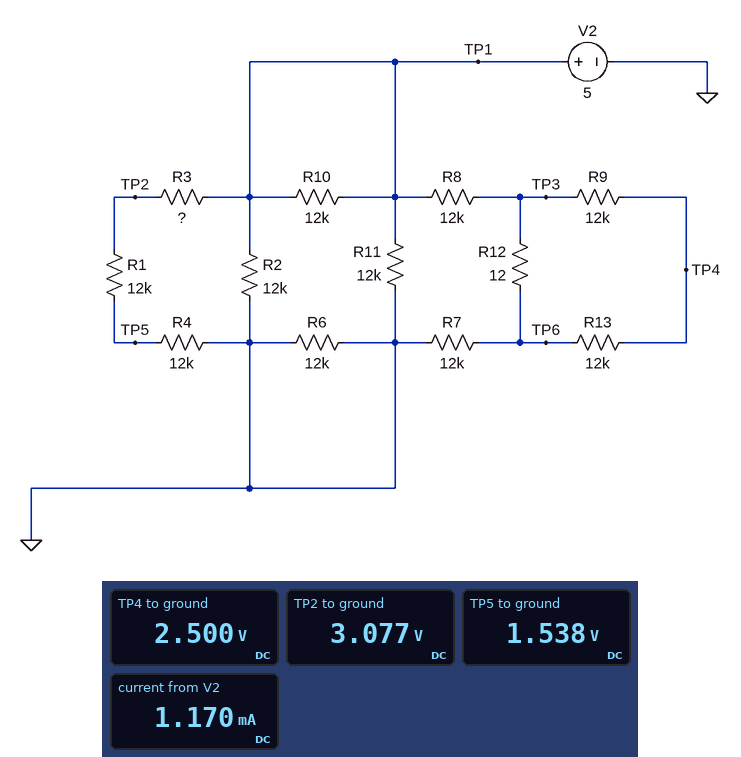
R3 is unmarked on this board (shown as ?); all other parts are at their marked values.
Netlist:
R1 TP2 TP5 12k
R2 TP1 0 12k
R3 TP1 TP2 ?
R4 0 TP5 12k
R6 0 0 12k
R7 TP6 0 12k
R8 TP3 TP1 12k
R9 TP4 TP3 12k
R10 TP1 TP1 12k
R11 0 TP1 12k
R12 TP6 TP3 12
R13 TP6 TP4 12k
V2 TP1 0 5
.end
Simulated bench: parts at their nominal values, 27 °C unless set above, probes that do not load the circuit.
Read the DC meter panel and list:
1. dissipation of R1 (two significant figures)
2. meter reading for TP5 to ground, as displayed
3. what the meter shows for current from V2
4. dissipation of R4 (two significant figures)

200 µW
1.538 V
1.170 mA
200 µW
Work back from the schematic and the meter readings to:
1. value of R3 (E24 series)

15 kΩ
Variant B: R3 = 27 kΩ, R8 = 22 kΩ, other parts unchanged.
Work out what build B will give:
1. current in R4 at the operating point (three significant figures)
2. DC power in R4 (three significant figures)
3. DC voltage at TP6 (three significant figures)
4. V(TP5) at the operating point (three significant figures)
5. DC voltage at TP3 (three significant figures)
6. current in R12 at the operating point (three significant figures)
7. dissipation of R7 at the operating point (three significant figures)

98.0 µA
115 µW
1.76 V
1.18 V
1.77 V
147 µA
259 µW
